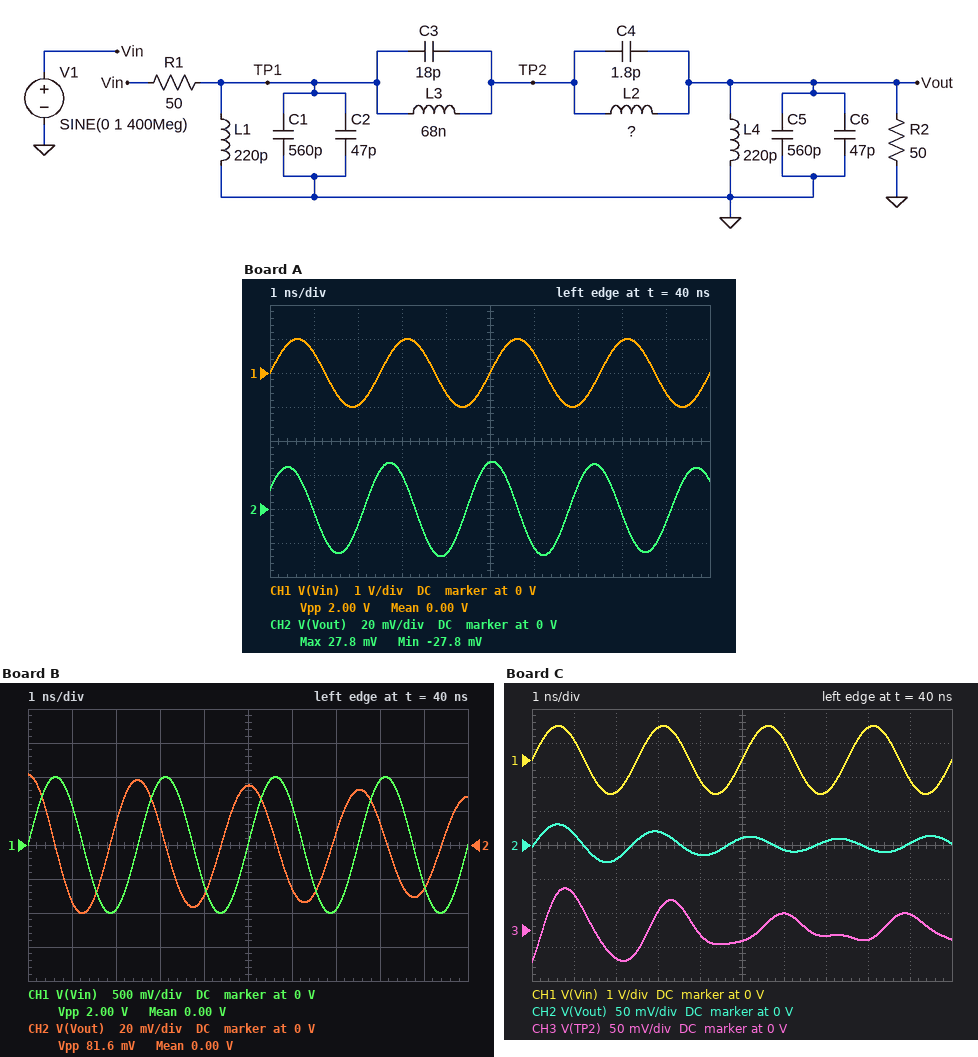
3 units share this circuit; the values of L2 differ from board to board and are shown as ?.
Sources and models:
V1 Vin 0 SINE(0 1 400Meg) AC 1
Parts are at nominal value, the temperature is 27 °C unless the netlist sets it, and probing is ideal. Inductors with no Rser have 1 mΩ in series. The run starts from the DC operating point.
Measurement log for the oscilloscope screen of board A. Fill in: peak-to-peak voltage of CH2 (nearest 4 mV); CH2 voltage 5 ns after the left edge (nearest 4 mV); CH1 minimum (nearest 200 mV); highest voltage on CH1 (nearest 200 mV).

56 mV
28 mV
-1.0 V
1.0 V
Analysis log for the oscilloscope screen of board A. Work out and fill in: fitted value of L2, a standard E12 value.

18 nH
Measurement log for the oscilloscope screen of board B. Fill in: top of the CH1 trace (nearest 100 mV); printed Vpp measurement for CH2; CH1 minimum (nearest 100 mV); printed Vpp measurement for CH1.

1.0 V
81.6 mV
-1.0 V
2.00 V
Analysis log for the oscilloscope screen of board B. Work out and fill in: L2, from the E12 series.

10 nH
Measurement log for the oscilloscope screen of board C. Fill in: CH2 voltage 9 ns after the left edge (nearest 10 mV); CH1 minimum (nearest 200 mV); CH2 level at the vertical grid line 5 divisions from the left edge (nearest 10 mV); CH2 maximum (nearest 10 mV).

0 V
-1.0 V
10 mV
30 mV
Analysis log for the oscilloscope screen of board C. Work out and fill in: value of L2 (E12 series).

2.7 nH
